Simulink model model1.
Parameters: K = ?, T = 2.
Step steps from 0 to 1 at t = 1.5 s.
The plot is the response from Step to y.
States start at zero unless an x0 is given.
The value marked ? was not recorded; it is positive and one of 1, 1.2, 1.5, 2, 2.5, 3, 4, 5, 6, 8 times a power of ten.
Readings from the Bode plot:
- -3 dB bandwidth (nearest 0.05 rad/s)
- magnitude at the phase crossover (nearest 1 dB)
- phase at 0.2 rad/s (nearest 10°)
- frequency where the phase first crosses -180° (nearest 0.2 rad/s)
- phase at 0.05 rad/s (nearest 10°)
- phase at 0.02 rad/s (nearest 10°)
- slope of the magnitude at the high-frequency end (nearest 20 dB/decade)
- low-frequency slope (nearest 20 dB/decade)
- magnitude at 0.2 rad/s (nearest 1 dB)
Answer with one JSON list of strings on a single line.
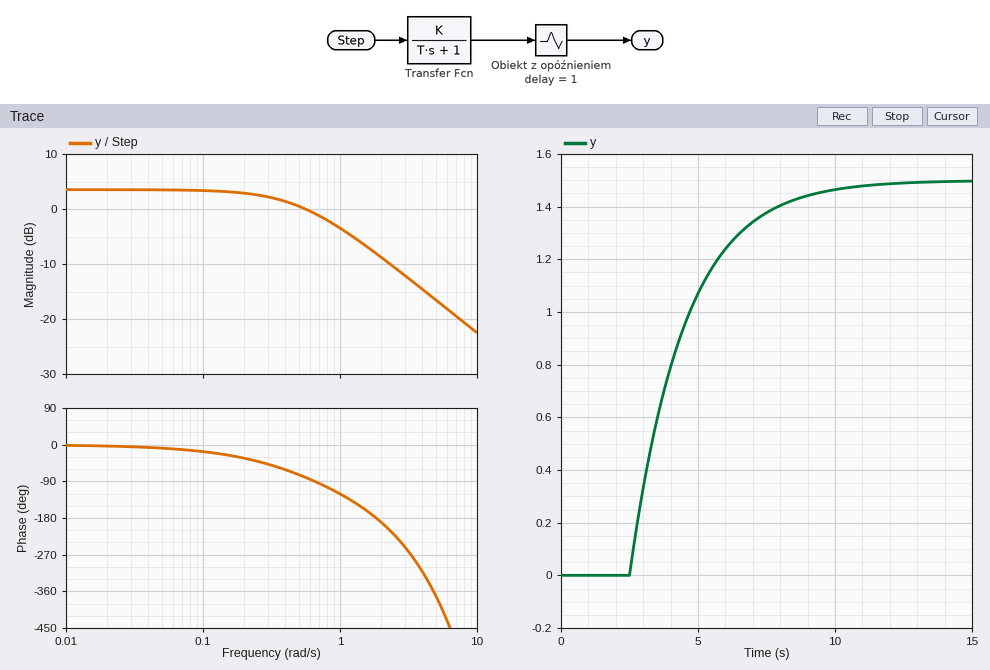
["0.50 rad/s", "-8 dB", "-30°", "1.8 rad/s", "-10°", "0°", "-20 dB/decade", "0 dB/decade", "3 dB"]
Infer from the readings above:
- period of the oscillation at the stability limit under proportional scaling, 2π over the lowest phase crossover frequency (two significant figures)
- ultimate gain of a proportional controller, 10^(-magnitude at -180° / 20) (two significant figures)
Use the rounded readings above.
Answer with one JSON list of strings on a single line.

["3.5 s", "2.5"]
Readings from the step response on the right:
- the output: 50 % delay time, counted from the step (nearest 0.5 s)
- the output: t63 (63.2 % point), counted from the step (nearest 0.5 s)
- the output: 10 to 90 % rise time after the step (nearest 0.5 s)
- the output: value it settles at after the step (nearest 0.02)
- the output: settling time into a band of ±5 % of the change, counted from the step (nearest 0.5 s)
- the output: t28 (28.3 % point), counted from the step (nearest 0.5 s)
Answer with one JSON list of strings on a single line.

["2.5 s", "3.0 s", "4.5 s", "1.50", "7.0 s", "1.5 s"]
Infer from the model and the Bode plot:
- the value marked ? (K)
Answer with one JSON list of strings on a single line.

["1.5"]
